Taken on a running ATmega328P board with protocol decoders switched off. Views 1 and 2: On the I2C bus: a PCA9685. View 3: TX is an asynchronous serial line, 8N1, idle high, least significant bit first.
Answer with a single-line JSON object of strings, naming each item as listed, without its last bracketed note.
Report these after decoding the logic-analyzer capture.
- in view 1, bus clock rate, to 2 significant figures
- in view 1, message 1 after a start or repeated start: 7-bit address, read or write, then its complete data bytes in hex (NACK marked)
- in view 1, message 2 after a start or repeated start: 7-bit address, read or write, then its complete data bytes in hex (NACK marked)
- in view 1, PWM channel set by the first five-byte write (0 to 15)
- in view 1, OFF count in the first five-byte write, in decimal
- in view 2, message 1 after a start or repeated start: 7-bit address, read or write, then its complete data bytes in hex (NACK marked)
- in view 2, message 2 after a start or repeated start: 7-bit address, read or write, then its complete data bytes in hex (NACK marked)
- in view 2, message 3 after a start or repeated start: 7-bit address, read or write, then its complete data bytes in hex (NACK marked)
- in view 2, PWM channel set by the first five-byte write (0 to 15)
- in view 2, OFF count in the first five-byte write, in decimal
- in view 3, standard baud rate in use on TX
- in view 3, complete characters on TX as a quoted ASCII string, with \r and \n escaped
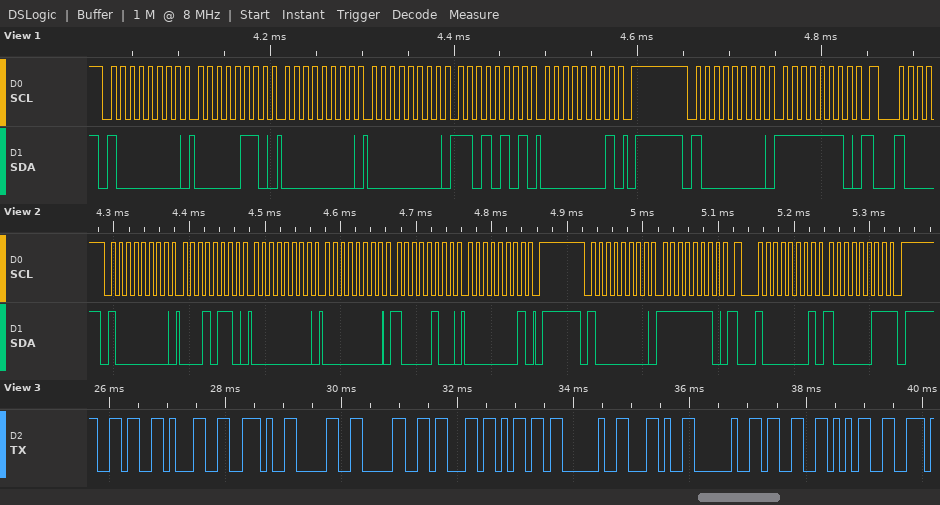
{"in view 1, bus clock rate, to 2 significant figures": "100 kHz", "in view 1, message 1 after a start or repeated start: 7-bit address, read or write, then its complete data bytes in hex": "0x40 write: 06 00 00 D5 01", "in view 1, message 2 after a start or repeated start: 7-bit address, read or write, then its complete data bytes in hex": "0x40 write: FE", "in view 1, PWM channel set by the first five-byte write": "0", "in view 1, OFF count in the first five-byte write, in decimal": "469", "in view 2, message 1 after a start or repeated start: 7-bit address, read or write, then its complete data bytes in hex": "0x40 write: 16 00 00 84 01", "in view 2, message 2 after a start or repeated start: 7-bit address, read or write, then its complete data bytes in hex": "0x40 write: FE", "in view 2, message 3 after a start or repeated start: 7-bit address, read or write, then its complete data bytes in hex": "0x40 read: 83 NACK", "in view 2, PWM channel set by the first five-byte write": "4", "in view 2, OFF count in the first five-byte write, in decimal": "388", "in view 3, standard baud rate in use on TX": "9600 baud", "in view 3, complete characters on TX as a quoted ASCII string, with \\r and \\n escaped": "\"61.00cm , 35\""}
